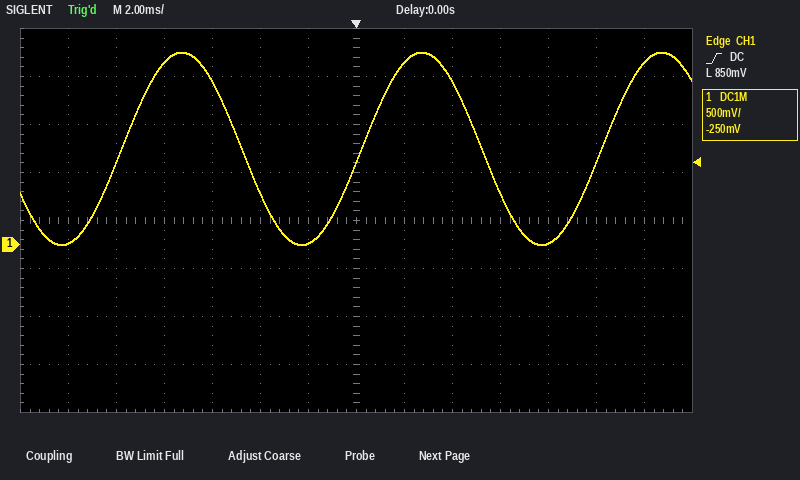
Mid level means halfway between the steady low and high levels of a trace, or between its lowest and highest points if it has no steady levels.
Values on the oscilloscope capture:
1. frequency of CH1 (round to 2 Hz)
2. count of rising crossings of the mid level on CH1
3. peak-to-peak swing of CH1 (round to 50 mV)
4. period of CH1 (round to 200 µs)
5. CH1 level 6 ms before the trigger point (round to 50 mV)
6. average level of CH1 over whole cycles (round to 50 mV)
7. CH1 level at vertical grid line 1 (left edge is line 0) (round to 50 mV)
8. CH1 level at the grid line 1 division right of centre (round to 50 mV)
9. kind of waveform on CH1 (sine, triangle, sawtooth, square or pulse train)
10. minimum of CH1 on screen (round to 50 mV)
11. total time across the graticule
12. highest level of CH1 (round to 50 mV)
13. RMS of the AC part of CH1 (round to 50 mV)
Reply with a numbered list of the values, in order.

1. 100 Hz
2. 3
3. 2.00 V
4. 10.0 ms
5. 1.70 V
6. 1.00 V
7. 0 mV
8. 1.90 V
9. sine
10. 0 mV
11. 28 ms
12. 2.00 V
13. 700 mV
